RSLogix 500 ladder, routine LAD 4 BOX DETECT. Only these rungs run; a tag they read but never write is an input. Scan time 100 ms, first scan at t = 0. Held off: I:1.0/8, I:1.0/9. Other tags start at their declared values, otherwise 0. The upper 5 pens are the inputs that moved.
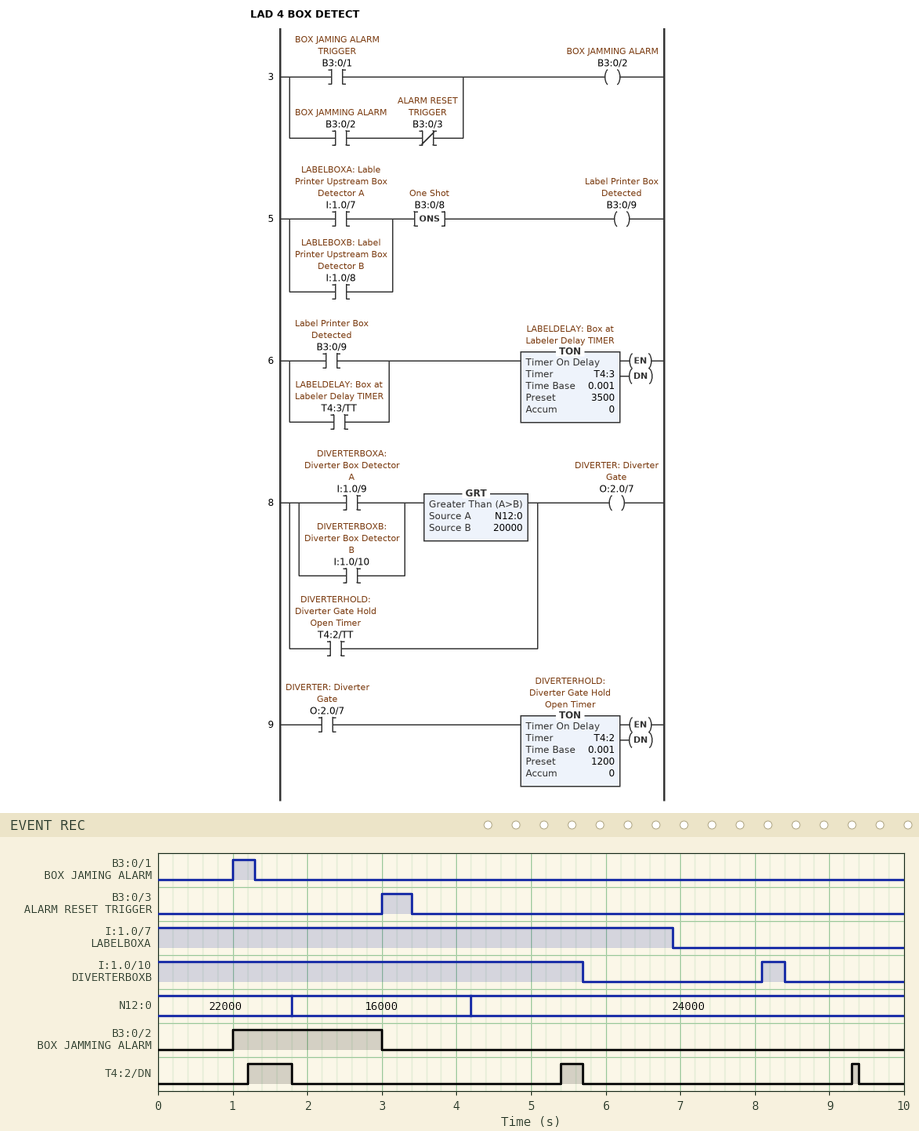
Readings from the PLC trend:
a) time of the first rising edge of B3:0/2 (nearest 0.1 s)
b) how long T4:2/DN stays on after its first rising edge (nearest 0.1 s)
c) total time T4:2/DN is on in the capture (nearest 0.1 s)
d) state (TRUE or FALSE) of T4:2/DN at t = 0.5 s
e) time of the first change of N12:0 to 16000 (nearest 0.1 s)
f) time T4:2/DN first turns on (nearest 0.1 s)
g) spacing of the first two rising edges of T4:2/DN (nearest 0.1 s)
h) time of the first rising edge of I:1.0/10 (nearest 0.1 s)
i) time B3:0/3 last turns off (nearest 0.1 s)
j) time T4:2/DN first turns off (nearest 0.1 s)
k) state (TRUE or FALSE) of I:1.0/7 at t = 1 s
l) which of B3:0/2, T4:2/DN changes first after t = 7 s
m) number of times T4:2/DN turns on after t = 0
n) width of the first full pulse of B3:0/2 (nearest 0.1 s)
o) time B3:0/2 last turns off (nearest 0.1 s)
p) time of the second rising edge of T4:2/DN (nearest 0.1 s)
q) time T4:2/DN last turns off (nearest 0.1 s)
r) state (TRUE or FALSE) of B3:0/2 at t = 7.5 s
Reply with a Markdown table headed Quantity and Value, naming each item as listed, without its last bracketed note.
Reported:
| Quantity | Value |
|---|---|
| time of the first rising edge of B3:0/2 | 1.0 s |
| how long T4:2/DN stays on after its first rising edge | 0.6 s |
| total time T4:2/DN is on in the capture | 1.0 s |
| state (TRUE or FALSE) of T4:2/DN at t = 0.5 s | FALSE |
| time of the first change of N12:0 to 16000 | 1.8 s |
| time T4:2/DN first turns on | 1.2 s |
| spacing of the first two rising edges of T4:2/DN | 4.2 s |
| time of the first rising edge of I:1.0/10 | 8.1 s |
| time B3:0/3 last turns off | 3.4 s |
| time T4:2/DN first turns off | 1.8 s |
| state (TRUE or FALSE) of I:1.0/7 at t = 1 s | TRUE |
| which of B3:0/2, T4:2/DN changes first after t = 7 s | T4:2/DN |
| number of times T4:2/DN turns on after t = 0 | 3 |
| width of the first full pulse of B3:0/2 | 2.0 s |
| time B3:0/2 last turns off | 3.0 s |
| time of the second rising edge of T4:2/DN | 5.4 s |
| time T4:2/DN last turns off | 9.4 s |
| state (TRUE or FALSE) of B3:0/2 at t = 7.5 s | FALSE |
